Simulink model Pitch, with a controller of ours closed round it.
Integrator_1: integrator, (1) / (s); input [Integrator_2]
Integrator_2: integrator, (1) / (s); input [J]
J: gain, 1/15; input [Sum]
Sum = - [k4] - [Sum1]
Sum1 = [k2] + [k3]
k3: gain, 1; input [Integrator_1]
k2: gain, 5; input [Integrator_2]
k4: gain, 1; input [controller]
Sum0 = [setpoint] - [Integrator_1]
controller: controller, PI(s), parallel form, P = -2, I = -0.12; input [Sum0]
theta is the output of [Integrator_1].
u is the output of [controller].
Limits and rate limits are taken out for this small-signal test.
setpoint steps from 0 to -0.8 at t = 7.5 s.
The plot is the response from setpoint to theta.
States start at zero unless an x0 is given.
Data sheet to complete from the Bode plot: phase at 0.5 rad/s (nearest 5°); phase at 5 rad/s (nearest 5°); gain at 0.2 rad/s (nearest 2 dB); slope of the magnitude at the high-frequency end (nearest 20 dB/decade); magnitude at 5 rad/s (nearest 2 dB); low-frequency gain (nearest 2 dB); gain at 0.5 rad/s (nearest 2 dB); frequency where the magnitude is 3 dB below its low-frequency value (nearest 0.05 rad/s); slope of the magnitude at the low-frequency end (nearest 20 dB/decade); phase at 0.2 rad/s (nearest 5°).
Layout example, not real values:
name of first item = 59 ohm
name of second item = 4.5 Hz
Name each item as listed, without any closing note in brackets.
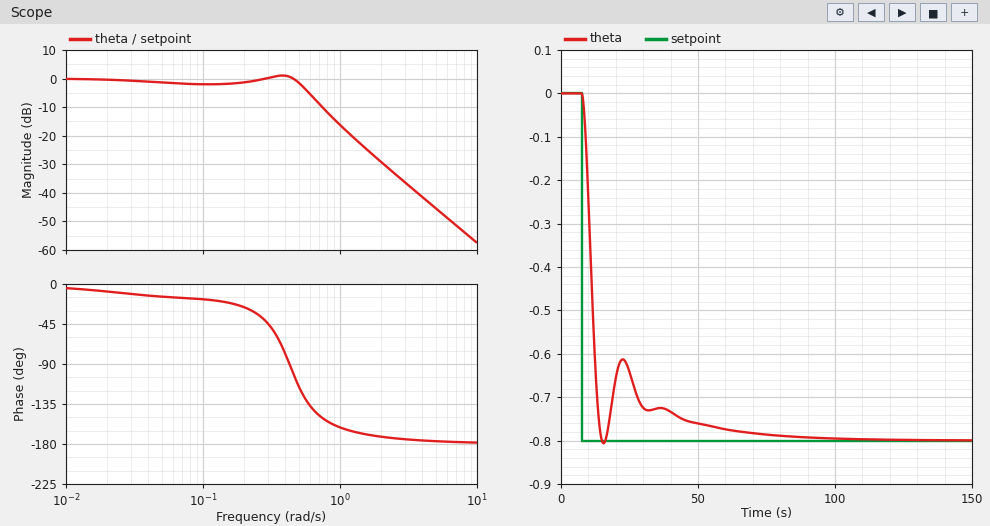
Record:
phase at 0.5 rad/s = -115°
phase at 5 rad/s = -175°
gain at 0.2 rad/s = -2 dB
slope of the magnitude at the high-frequency end = -40 dB/decade
magnitude at 5 rad/s = -46 dB
low-frequency gain = 0 dB
gain at 0.5 rad/s = -2 dB
frequency where the magnitude is 3 dB below its low-frequency value = 0.55 rad/s
slope of the magnitude at the low-frequency end = 0 dB/decade
phase at 0.2 rad/s = -25°
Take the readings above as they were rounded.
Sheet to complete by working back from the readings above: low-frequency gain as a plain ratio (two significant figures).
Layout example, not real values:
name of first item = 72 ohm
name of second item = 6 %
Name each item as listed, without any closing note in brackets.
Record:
low-frequency gain as a plain ratio = 1.0
